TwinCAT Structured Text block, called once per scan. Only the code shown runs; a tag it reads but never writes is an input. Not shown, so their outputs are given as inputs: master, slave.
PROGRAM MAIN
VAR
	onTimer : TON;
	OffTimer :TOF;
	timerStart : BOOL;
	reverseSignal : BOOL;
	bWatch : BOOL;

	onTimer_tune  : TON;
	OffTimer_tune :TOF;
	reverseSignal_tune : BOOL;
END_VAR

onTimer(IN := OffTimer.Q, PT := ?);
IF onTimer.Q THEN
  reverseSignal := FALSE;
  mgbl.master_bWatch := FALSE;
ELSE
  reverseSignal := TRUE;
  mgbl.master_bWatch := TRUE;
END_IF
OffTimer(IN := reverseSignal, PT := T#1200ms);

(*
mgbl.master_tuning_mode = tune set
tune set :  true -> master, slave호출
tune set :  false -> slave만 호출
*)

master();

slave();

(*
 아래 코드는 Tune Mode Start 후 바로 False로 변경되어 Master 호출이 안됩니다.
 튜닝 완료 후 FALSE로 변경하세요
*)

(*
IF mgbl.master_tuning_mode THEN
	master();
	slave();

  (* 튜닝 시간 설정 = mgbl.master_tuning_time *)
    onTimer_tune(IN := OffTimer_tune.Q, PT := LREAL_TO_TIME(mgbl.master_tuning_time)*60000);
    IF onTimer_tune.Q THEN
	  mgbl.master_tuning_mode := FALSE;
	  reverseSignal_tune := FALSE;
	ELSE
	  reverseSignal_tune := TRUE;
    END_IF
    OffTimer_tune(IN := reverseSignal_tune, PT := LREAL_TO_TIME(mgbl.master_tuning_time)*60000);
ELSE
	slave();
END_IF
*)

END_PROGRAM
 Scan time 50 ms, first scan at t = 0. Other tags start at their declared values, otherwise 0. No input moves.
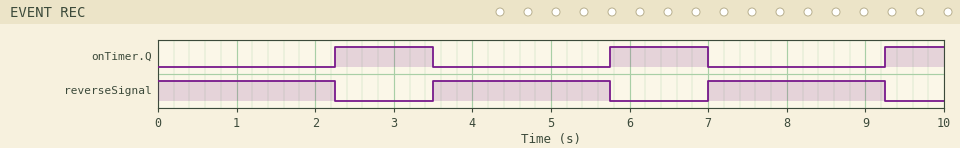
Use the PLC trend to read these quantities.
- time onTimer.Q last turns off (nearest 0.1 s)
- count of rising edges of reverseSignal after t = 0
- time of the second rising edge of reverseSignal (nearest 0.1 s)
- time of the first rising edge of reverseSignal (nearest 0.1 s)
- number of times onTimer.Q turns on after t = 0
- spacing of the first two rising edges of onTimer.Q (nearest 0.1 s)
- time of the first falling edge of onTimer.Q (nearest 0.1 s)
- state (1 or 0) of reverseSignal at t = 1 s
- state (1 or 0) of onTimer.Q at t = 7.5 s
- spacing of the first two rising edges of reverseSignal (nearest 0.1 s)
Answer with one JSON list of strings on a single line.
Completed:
["7.0 s", "2", "7.0 s", "3.5 s", "3", "3.5 s", "3.5 s", "1", "0", "3.5 s"]
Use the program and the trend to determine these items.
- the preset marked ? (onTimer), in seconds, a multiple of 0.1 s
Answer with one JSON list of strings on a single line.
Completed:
["2.2 s"]
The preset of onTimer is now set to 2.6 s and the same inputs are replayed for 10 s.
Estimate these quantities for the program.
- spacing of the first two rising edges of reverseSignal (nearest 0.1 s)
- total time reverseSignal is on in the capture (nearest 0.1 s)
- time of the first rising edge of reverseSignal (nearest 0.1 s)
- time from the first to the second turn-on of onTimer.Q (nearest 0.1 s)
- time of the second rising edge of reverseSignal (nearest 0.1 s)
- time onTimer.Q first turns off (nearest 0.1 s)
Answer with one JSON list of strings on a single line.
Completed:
["3.9 s", "7.5 s", "3.9 s", "3.9 s", "7.8 s", "3.9 s"]
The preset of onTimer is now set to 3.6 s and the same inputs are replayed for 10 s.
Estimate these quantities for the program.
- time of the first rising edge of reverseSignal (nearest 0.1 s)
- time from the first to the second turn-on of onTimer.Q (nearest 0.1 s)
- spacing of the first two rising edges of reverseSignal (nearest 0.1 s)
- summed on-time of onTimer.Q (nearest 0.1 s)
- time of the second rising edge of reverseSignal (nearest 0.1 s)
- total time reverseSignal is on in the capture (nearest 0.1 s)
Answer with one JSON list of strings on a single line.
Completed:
["4.9 s", "4.9 s", "4.9 s", "2.5 s", "9.8 s", "7.5 s"]
